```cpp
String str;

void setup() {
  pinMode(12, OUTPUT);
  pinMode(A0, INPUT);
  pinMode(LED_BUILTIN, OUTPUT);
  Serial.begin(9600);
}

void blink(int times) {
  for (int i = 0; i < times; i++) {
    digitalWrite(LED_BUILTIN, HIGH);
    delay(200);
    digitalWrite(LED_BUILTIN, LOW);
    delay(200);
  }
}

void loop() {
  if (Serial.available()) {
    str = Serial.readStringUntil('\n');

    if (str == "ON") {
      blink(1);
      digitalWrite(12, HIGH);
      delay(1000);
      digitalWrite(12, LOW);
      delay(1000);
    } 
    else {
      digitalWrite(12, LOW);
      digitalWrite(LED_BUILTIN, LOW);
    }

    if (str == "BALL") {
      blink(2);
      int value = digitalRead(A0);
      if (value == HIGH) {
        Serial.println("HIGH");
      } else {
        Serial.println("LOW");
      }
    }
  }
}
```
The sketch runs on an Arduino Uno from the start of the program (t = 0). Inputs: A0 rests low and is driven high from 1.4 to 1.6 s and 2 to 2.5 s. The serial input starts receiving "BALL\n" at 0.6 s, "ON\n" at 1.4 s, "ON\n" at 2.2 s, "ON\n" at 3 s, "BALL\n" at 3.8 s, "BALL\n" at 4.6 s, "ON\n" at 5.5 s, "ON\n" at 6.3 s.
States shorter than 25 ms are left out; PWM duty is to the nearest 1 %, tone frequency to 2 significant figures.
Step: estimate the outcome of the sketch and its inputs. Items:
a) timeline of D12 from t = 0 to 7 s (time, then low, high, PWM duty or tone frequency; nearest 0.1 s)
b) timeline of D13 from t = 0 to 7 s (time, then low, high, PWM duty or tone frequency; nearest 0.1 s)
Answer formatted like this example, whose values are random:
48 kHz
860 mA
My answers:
0 s low; 1.8 s high; 2.8 s low; 4.2 s high; 5.2 s low; 6.6 s high
0 s low; 0.6 s high; 0.8 s low; 1 s high; 1.2 s low; 1.4 s high; 1.6 s low; 3.8 s high; 4 s low; 6.2 s high; 6.4 s low
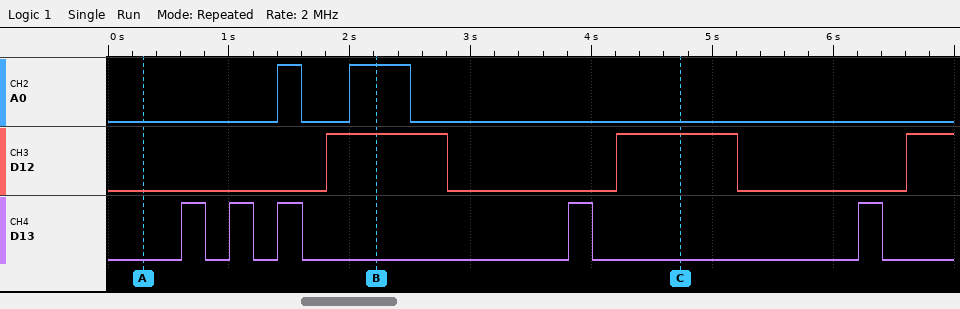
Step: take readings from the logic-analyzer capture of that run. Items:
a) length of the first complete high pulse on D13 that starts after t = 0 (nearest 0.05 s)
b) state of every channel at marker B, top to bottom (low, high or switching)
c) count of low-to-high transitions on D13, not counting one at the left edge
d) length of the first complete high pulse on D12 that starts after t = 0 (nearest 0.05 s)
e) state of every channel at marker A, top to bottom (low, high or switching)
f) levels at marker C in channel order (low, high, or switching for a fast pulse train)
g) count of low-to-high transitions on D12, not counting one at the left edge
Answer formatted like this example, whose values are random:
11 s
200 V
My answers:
0.20 s
A0 high, D12 high, D13 low
5
1.00 s
A0 low, D12 low, D13 low
A0 low, D12 high, D13 low
3
